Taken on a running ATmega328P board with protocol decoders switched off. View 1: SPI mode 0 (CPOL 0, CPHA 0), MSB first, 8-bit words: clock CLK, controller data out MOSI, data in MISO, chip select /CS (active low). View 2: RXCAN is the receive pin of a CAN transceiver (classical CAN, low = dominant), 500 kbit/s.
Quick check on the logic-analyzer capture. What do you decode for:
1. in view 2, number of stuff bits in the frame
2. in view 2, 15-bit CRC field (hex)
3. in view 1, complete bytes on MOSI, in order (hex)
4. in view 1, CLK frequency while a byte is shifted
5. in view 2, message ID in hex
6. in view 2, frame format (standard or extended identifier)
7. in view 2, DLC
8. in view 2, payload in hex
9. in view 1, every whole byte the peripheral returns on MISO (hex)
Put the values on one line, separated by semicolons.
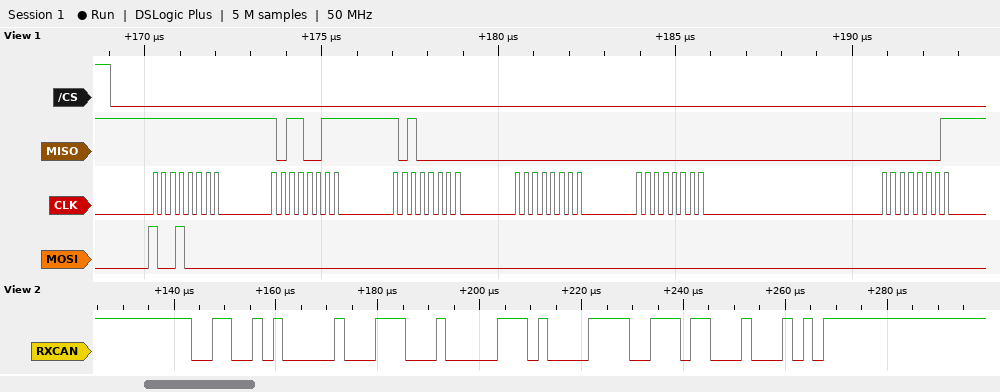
2; 0x7622; 90 00 00 00 00 00; 4 MHz; 0x328; standard; 3; 88 34 3C; FF B3 A0 00 00 01
